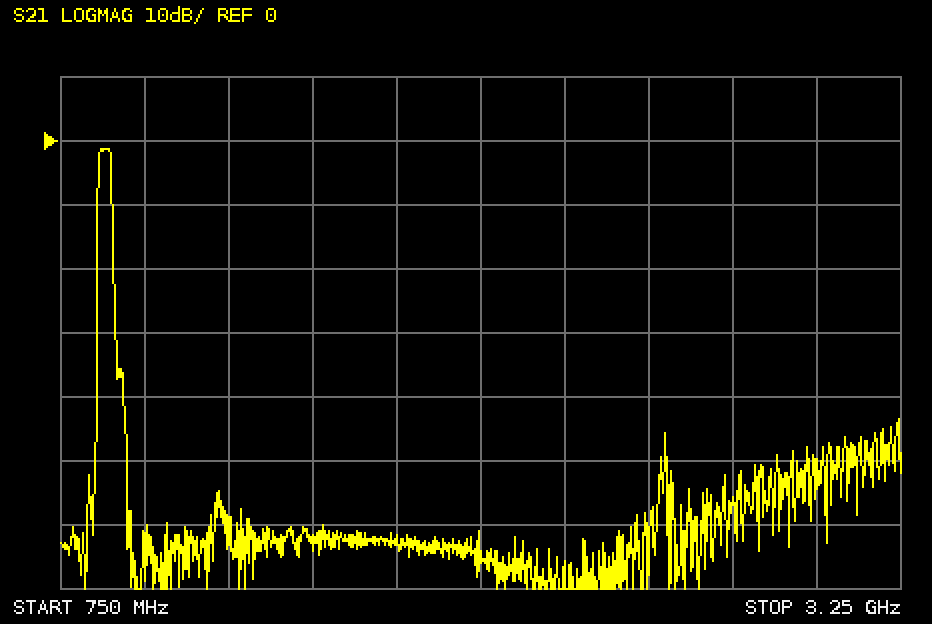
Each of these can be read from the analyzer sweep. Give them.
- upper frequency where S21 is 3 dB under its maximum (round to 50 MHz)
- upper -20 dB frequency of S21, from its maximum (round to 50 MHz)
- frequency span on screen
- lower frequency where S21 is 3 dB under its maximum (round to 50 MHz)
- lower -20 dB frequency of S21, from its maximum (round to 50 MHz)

900 MHz
900 MHz
2.5 GHz
850 MHz
850 MHz
